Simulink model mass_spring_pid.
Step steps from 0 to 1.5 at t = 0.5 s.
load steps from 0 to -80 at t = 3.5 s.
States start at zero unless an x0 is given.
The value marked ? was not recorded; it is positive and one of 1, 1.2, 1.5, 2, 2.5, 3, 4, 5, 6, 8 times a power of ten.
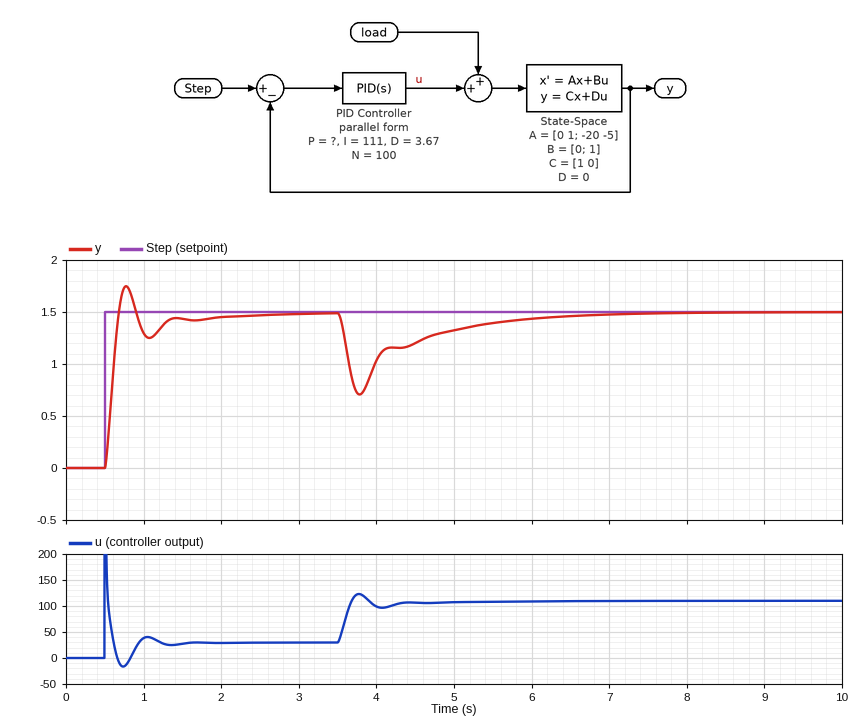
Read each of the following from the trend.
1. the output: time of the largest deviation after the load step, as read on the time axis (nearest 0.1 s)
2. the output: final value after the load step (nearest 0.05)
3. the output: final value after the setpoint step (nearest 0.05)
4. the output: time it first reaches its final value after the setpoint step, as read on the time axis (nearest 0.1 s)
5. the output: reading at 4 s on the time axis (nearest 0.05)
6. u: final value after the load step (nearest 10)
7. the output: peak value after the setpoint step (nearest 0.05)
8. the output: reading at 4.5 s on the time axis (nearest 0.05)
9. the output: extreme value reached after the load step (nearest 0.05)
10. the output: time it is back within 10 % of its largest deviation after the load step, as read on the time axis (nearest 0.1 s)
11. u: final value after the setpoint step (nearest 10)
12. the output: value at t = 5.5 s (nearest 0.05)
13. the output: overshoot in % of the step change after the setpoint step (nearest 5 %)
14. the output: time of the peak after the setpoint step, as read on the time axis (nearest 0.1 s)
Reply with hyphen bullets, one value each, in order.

- 3.8 s
- 1.50
- 1.50
- 0.7 s
- 1.05
- 110
- 1.75
- 1.20
- 0.70
- 5.8 s
- 30
- 1.40
- 15 %
- 0.8 s
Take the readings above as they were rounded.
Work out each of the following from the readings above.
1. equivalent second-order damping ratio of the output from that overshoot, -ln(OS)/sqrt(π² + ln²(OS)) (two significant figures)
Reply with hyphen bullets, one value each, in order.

- 0.52
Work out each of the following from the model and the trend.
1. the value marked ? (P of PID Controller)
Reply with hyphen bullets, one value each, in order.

- 100
